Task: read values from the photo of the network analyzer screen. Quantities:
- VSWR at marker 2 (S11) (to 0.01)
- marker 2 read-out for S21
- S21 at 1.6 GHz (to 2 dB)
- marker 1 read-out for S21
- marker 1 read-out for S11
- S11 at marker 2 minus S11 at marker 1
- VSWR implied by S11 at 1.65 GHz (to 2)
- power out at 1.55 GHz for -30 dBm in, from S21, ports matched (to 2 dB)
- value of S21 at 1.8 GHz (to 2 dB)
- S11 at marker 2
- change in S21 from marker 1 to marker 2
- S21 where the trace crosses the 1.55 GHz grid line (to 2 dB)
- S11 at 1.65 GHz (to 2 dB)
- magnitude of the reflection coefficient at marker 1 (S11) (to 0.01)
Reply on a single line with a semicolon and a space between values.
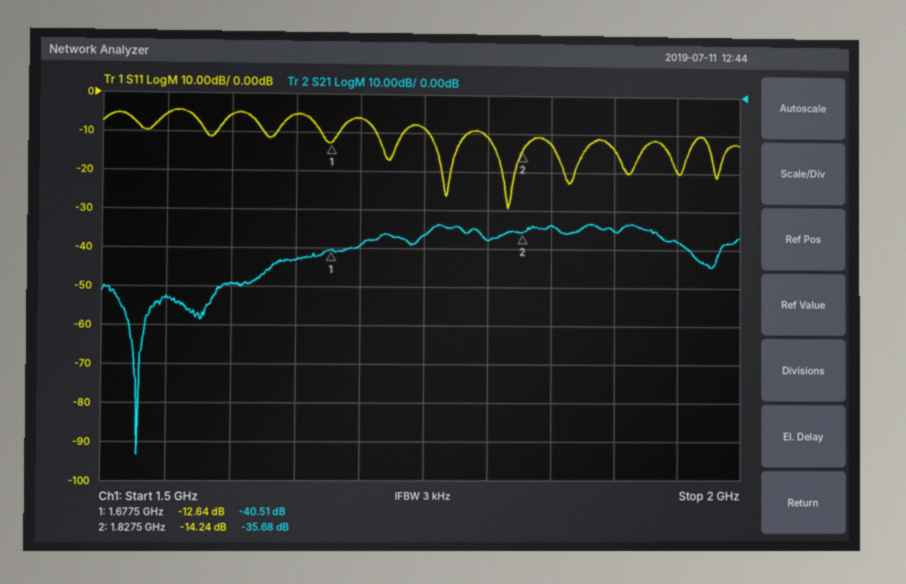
1.48; -35.68 dB; -50 dB; -40.51 dB; -12.64 dB; -1.60 dB; 4; -82 dBm; -38 dB; -14.24 dB; 4.83 dB; -52 dB; -6 dB; 0.23
